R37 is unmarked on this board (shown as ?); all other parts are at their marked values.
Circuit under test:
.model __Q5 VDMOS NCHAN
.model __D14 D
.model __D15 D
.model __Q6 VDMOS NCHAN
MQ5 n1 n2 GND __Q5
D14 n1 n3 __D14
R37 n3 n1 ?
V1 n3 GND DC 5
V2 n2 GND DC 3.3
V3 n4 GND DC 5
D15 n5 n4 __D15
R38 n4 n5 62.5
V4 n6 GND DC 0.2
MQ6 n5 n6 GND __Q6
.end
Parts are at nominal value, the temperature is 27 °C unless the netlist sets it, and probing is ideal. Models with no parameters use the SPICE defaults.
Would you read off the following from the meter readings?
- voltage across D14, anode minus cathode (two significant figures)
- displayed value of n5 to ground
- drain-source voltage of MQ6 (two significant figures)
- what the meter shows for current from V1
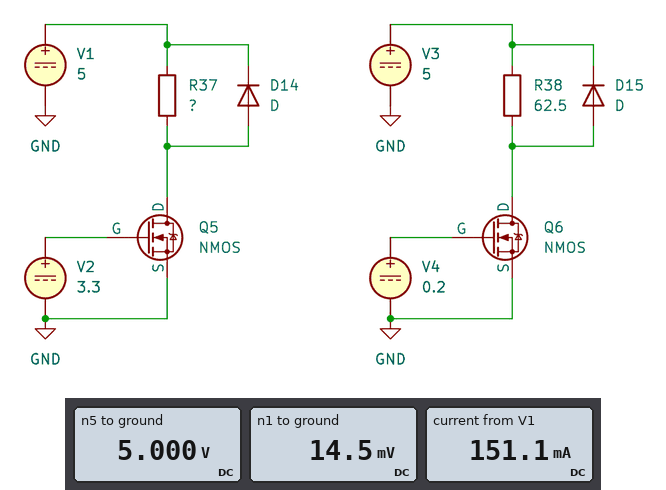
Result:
-5.0 V
5.000 V
5.0 V
151.1 mA
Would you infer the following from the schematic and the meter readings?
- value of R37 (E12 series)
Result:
33 Ω
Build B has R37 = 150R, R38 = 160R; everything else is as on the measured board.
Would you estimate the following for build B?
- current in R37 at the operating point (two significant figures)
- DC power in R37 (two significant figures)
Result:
33 mA
170 mW
